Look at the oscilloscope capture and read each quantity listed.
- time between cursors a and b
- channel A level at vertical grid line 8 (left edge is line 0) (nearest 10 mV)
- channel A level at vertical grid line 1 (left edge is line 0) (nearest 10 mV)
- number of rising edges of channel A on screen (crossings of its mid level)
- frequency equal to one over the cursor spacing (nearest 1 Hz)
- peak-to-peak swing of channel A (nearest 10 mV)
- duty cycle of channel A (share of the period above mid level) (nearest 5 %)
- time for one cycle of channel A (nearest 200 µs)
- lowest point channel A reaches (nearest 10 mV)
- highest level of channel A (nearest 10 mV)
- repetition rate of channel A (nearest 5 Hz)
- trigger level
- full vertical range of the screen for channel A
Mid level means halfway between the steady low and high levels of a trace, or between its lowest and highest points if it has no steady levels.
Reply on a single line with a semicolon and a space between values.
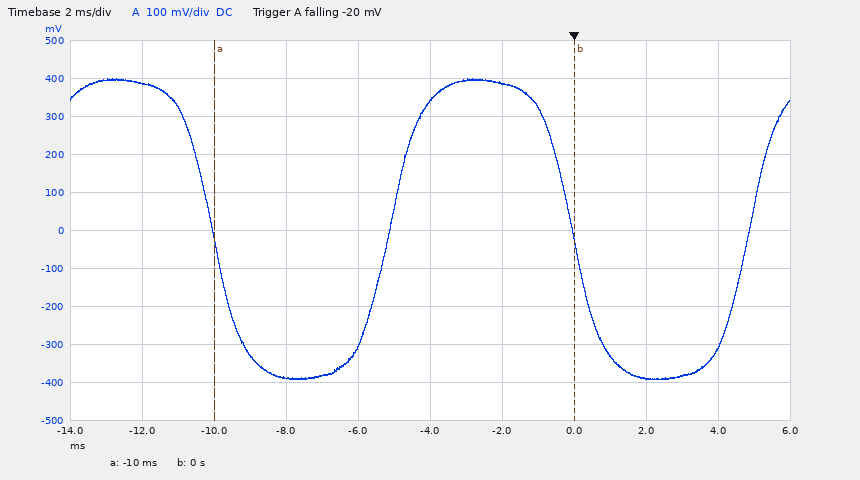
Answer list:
10.0 ms; -390 mV; 390 mV; 2; 100 Hz; 790 mV; 50 %; 10.0 ms; -390 mV; 400 mV; 100 Hz; -20 mV; 1 V
